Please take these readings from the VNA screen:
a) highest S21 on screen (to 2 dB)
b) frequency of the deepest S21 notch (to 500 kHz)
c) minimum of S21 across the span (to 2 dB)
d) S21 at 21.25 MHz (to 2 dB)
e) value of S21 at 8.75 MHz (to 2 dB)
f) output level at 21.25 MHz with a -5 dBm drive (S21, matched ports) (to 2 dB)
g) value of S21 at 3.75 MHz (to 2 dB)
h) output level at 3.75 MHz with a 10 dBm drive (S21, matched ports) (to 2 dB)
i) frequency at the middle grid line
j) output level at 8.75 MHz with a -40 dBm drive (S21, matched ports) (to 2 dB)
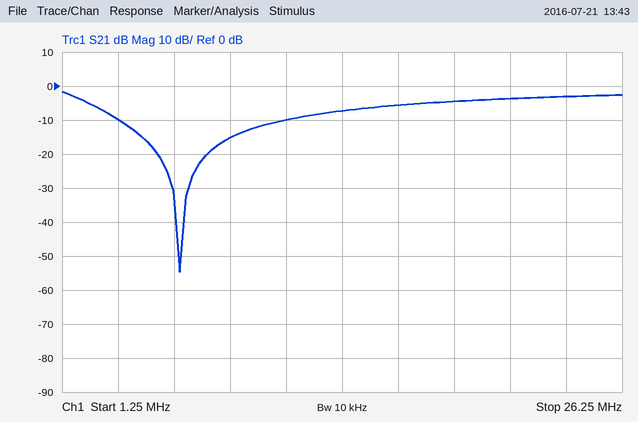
-2 dB
6.5 MHz
-54 dB
-4 dB
-16 dB
-8 dBm
-10 dB
0 dBm
13.75 MHz
-56 dBm
